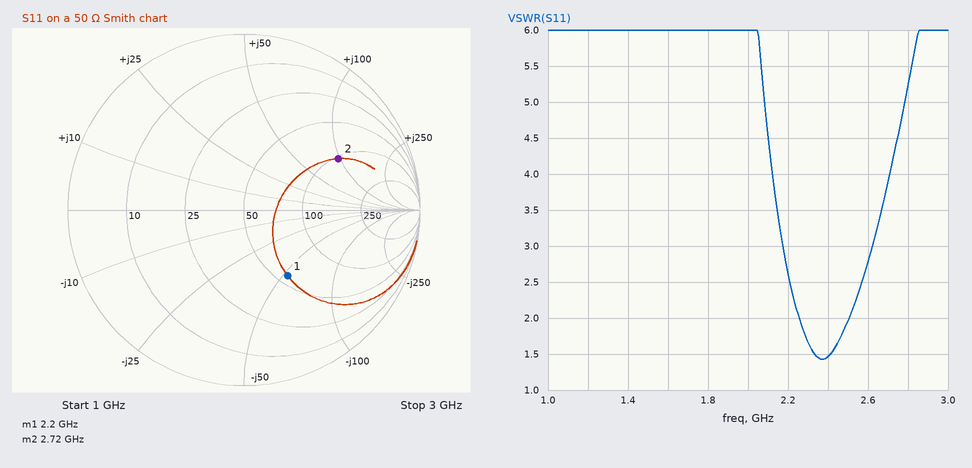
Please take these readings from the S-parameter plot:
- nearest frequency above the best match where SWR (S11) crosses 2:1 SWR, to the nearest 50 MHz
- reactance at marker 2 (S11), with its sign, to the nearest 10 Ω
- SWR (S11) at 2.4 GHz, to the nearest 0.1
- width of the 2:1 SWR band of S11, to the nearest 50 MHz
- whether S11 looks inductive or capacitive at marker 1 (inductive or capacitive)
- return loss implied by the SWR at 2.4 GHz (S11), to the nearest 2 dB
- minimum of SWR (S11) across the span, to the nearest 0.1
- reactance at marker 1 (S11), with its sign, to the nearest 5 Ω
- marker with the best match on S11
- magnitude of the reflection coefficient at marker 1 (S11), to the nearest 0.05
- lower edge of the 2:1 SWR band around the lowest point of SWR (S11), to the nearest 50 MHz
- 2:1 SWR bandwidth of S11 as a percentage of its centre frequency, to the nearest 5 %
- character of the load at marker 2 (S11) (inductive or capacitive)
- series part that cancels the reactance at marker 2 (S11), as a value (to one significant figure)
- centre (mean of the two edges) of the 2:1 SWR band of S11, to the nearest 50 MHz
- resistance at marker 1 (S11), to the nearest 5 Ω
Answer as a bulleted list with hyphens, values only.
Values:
- 2.50 GHz
- +100 Ω
- 1.5
- 250 MHz
- capacitive
- 14 dB
- 1.4
- -55 Ω
- marker 1
- 0.45
- 2.25 GHz
- 10 %
- inductive
- 600 fF
- 2.40 GHz
- 55 Ω
